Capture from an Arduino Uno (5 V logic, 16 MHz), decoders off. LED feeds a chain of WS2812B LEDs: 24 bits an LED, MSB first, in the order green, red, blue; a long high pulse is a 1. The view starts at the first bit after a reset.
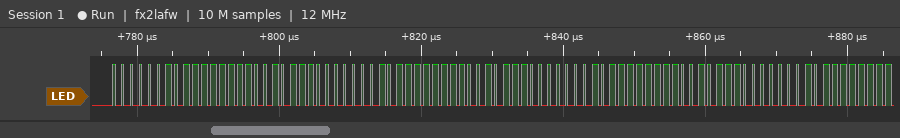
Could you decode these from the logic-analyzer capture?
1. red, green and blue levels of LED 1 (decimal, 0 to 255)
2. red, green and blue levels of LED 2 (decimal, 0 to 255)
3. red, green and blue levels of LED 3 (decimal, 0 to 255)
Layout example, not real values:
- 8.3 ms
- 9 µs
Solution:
- 255, 2, 46
- 255, 2, 46
- 255, 2, 46
